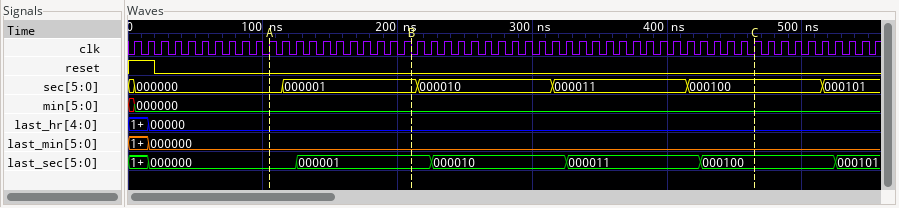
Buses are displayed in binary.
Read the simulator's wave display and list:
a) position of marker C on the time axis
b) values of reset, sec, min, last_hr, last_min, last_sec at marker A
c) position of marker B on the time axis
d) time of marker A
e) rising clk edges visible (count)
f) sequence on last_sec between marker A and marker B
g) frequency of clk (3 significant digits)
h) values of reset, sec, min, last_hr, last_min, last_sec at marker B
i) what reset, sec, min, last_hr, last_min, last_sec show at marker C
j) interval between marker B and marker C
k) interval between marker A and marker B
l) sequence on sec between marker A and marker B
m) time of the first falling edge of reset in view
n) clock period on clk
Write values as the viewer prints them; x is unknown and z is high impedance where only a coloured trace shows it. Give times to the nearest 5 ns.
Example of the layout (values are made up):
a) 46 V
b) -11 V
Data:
a) 465 ns
b) reset=0, sec=000000, min=000000, last_hr=00000, last_min=000000, last_sec=000000
c) 210 ns
d) 105 ns
e) 56
f) 000000, 000001
g) 100 MHz
h) reset=0, sec=000001, min=000000, last_hr=00000, last_min=000000, last_sec=000001
i) reset=0, sec=000100, min=000000, last_hr=00000, last_min=000000, last_sec=000100
j) 255 ns
k) 105 ns
l) 000000, 000001
m) 20 ns
n) 10 ns
